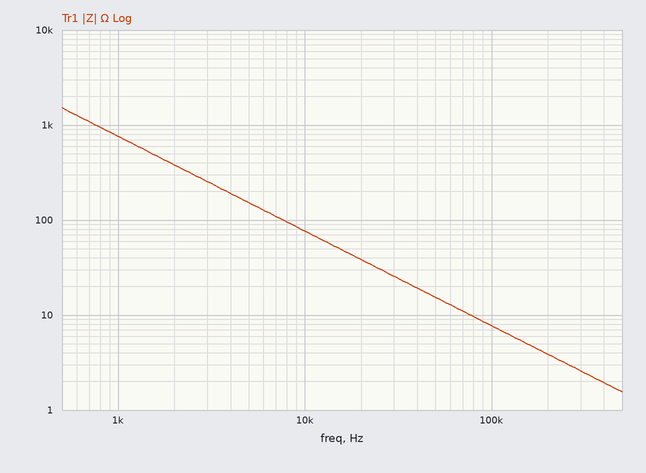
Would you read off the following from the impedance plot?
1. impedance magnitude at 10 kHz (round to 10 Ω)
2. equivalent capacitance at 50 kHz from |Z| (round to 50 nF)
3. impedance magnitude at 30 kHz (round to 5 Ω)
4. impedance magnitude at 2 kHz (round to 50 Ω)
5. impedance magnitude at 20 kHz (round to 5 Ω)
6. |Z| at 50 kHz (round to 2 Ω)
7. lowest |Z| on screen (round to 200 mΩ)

80 Ω
200 nF
25 Ω
400 Ω
40 Ω
16 Ω
1.6 Ω
